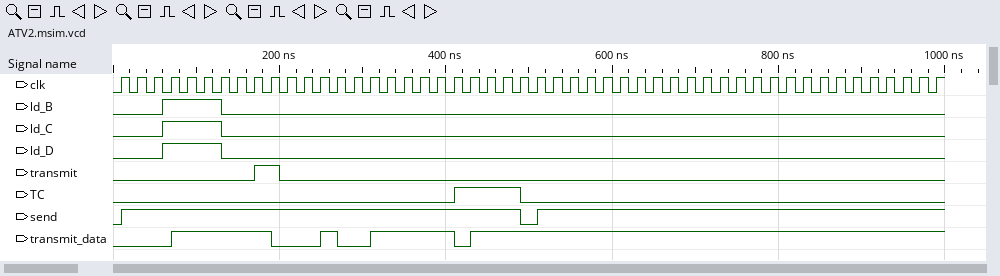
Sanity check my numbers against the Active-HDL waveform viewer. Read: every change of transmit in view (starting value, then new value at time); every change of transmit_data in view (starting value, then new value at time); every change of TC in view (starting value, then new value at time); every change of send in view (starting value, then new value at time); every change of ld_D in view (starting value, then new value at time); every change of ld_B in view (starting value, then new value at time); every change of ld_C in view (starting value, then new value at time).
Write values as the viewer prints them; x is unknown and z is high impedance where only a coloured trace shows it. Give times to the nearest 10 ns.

0, 1 at 170 ns, 0 at 200 ns
0, 1 at 70 ns, 0 at 190 ns, 1 at 250 ns, 0 at 270 ns, 1 at 310 ns, 0 at 410 ns, 1 at 430 ns
0, 1 at 410 ns, 0 at 490 ns
0, 1 at 10 ns, 0 at 490 ns, 1 at 510 ns
0, 1 at 60 ns, 0 at 130 ns
0, 1 at 60 ns, 0 at 130 ns
0, 1 at 60 ns, 0 at 130 ns
